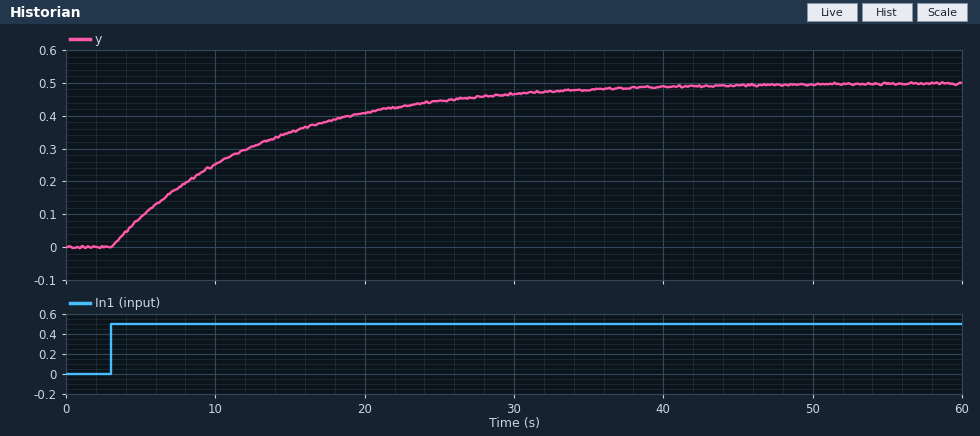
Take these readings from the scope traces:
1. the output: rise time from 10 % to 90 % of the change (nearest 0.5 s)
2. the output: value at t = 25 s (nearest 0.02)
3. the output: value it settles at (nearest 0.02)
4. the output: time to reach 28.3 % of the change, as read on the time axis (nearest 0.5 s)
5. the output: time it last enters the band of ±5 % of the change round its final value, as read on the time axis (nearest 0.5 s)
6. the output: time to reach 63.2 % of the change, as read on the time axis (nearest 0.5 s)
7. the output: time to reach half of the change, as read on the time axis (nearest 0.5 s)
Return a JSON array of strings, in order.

["22.0 s", "0.44", "0.50", "6.5 s", "33.0 s", "13.0 s", "10.0 s"]
